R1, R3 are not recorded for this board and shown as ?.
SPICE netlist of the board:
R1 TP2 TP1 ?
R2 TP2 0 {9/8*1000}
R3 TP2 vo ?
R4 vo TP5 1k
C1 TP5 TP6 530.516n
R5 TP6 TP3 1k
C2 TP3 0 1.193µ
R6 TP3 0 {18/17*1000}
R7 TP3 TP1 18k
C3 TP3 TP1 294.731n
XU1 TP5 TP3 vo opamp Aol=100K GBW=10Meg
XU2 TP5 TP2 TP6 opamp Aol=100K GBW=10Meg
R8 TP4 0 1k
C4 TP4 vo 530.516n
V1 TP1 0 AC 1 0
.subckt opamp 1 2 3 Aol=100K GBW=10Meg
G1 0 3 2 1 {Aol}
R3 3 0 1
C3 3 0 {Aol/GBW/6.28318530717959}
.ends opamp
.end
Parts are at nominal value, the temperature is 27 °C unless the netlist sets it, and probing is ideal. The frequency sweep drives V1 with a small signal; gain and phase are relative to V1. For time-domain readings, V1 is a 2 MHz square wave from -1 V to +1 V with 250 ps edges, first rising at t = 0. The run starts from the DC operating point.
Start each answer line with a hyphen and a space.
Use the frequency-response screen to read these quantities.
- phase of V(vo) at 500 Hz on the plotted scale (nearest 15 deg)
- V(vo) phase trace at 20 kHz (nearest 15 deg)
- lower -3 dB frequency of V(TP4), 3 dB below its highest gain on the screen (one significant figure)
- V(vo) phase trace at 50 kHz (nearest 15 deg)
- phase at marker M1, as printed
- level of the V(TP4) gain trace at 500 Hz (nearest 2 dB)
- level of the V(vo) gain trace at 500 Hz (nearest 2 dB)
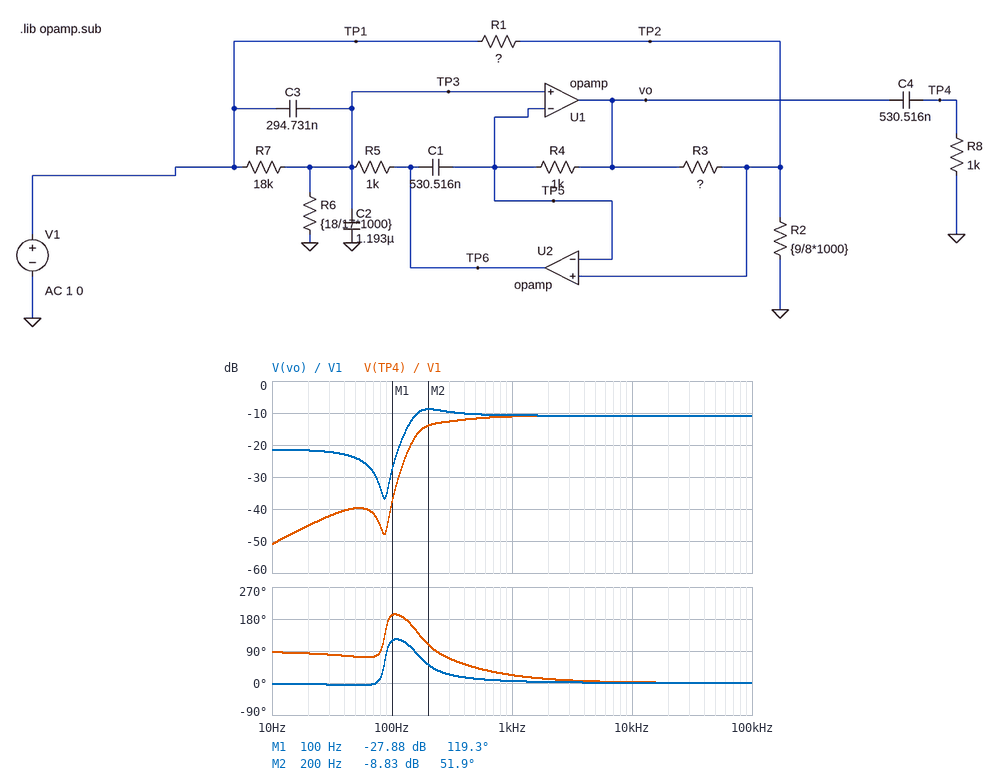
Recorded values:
- 15 deg
- 0 deg
- 200 Hz
- 0 deg
- 119.3 deg
- -12 dB
- -10 dB
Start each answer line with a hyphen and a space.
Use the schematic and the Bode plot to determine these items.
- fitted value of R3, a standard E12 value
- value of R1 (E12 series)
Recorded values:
- 820 Ω
- 12 kΩ
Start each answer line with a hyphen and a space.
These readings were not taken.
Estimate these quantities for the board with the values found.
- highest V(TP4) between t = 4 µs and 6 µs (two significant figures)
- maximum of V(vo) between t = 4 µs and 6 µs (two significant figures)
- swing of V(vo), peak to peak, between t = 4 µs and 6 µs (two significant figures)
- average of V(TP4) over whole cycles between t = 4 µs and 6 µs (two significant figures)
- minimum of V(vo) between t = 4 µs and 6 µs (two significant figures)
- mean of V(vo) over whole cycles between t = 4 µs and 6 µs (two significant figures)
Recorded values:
- 640 mV
- 560 mV
- 710 mV
- 280 mV
- -160 mV
- 200 mV
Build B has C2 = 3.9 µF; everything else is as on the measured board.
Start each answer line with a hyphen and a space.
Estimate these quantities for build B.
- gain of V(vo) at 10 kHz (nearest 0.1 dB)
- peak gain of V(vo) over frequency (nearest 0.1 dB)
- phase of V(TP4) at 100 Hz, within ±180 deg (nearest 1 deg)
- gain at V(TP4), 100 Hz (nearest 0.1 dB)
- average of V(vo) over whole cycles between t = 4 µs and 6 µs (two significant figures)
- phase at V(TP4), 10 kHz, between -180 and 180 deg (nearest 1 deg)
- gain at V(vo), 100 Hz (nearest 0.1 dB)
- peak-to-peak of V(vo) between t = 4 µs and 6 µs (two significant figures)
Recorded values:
- -24.7 dB
- -19.7 dB
- -1 deg
- -34.5 dB
- -28 mV
- 2 deg
- -24.5 dB
- 190 mV
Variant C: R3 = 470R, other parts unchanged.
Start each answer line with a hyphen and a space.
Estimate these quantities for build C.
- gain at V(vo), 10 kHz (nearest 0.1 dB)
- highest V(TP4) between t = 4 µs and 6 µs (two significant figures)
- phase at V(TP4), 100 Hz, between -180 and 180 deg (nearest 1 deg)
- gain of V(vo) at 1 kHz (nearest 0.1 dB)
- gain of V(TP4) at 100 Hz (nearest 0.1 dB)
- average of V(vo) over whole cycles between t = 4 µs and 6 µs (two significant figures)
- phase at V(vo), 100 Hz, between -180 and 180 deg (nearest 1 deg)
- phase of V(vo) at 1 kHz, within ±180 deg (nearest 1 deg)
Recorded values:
- -12.1 dB
- 590 mV
- 165 deg
- -12.0 dB
- -29.0 dB
- 160 mV
- 94 deg
- 5 deg
